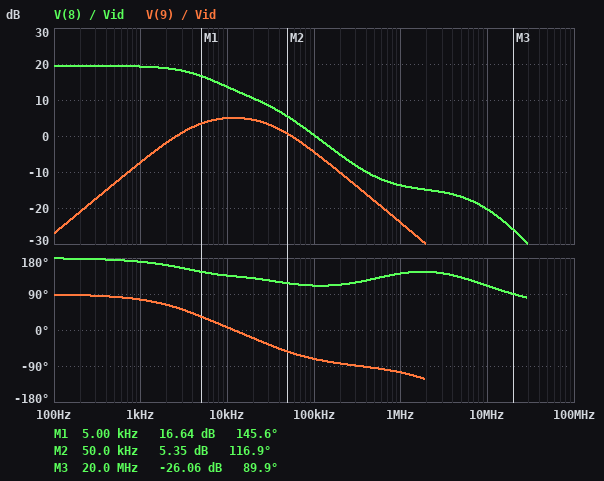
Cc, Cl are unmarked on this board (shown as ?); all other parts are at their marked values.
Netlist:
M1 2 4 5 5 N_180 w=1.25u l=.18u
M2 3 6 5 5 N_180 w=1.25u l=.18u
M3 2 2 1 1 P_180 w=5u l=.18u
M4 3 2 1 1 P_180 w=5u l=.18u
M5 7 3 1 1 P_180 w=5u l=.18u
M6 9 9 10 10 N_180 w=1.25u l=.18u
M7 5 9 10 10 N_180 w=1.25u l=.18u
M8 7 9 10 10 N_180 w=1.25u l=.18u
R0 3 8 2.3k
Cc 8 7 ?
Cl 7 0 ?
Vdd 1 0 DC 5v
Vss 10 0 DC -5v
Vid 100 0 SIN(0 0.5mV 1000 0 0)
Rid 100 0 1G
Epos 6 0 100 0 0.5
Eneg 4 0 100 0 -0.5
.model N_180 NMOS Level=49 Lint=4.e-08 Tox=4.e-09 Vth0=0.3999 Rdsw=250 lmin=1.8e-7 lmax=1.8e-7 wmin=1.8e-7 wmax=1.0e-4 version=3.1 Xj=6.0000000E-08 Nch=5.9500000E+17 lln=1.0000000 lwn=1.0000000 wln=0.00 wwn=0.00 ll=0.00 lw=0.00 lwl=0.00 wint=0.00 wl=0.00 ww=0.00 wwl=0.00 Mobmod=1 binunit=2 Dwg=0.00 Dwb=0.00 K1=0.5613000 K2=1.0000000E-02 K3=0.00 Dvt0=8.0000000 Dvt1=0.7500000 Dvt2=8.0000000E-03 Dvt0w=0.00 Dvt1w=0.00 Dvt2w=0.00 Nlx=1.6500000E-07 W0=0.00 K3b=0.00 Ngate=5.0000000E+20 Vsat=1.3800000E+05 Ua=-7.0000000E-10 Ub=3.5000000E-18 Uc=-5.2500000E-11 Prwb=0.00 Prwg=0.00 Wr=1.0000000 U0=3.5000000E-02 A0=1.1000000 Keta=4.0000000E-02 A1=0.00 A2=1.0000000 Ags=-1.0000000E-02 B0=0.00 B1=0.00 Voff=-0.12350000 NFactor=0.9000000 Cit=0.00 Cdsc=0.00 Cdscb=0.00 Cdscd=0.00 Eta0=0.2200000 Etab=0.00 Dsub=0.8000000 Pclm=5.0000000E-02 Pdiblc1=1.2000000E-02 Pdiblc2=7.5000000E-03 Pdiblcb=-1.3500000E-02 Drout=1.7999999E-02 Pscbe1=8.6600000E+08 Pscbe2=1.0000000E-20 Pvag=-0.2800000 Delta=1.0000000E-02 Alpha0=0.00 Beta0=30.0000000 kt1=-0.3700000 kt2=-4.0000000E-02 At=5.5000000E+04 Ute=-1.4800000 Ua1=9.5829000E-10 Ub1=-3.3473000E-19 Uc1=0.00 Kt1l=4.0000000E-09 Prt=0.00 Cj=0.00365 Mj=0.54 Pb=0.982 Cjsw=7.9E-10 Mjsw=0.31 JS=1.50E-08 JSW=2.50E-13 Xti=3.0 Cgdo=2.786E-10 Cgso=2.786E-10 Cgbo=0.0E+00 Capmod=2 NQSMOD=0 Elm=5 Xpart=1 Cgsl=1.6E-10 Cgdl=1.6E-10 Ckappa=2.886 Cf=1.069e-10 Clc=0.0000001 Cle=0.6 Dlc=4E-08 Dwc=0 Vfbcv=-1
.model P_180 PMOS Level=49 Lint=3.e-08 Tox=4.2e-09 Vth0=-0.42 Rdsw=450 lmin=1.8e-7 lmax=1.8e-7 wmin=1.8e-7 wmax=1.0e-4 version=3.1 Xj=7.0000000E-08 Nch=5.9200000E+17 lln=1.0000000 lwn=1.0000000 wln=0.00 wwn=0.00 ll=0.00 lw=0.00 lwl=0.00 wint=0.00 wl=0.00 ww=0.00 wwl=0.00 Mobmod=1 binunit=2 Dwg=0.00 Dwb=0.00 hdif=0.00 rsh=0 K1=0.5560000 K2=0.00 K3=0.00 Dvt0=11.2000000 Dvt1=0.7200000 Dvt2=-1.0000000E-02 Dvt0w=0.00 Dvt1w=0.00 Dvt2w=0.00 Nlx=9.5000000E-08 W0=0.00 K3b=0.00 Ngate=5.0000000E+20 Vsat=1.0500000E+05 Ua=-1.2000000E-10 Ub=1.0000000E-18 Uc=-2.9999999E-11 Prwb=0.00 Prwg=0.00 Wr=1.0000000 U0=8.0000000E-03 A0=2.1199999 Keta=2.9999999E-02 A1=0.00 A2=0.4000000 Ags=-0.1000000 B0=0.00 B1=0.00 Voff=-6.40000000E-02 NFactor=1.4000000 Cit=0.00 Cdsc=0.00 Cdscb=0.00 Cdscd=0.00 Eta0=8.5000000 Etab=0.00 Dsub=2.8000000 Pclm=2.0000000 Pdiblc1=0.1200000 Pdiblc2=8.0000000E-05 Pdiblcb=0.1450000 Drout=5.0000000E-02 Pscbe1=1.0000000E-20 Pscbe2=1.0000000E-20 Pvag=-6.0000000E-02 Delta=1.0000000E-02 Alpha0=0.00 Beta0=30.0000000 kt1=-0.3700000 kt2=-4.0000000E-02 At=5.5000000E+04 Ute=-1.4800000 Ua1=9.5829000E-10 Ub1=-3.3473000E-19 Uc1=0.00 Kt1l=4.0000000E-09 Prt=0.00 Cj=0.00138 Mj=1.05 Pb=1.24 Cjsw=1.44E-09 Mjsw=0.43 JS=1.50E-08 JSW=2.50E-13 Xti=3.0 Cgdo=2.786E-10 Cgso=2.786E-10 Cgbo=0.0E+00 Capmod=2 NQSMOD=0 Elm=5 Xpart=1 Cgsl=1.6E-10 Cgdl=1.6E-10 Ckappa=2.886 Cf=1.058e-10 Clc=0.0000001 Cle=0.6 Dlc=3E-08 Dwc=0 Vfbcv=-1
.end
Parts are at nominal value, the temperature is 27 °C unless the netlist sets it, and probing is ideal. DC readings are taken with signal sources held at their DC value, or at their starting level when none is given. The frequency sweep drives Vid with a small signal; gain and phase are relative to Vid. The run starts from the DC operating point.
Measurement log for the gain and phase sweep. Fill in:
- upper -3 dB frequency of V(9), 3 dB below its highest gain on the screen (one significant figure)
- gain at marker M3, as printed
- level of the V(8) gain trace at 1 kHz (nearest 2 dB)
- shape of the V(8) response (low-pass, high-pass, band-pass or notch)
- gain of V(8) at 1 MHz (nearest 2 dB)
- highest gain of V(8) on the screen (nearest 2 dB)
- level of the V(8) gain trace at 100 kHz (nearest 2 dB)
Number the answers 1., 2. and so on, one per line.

1. 40 kHz
2. -26.06 dB
3. 20 dB
4. low-pass
5. -14 dB
6. 20 dB
7. 0 dB
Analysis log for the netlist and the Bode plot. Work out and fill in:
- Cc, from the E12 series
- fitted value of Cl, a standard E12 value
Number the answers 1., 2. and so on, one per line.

1. 1.2 pF
2. 1.2 pF
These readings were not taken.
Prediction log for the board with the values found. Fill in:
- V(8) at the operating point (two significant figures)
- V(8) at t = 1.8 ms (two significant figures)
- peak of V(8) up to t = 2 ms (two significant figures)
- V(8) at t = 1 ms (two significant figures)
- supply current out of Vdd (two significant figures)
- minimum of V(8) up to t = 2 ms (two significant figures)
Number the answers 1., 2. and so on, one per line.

1. 4.8 V
2. 4.8 V
3. 4.8 V
4. 4.8 V
5. 2.1 µA
6. 4.8 V
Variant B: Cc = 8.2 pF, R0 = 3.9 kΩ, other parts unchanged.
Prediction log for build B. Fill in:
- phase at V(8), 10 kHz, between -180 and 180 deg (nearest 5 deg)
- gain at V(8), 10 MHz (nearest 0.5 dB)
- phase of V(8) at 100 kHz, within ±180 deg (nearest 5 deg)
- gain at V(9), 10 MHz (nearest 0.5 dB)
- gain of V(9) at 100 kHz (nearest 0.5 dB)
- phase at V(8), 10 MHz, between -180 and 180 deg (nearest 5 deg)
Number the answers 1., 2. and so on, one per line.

1. 120 deg
2. -26.0 dB
3. 130 deg
4. -47.5 dB
5. -21.0 dB
6. 115 deg
